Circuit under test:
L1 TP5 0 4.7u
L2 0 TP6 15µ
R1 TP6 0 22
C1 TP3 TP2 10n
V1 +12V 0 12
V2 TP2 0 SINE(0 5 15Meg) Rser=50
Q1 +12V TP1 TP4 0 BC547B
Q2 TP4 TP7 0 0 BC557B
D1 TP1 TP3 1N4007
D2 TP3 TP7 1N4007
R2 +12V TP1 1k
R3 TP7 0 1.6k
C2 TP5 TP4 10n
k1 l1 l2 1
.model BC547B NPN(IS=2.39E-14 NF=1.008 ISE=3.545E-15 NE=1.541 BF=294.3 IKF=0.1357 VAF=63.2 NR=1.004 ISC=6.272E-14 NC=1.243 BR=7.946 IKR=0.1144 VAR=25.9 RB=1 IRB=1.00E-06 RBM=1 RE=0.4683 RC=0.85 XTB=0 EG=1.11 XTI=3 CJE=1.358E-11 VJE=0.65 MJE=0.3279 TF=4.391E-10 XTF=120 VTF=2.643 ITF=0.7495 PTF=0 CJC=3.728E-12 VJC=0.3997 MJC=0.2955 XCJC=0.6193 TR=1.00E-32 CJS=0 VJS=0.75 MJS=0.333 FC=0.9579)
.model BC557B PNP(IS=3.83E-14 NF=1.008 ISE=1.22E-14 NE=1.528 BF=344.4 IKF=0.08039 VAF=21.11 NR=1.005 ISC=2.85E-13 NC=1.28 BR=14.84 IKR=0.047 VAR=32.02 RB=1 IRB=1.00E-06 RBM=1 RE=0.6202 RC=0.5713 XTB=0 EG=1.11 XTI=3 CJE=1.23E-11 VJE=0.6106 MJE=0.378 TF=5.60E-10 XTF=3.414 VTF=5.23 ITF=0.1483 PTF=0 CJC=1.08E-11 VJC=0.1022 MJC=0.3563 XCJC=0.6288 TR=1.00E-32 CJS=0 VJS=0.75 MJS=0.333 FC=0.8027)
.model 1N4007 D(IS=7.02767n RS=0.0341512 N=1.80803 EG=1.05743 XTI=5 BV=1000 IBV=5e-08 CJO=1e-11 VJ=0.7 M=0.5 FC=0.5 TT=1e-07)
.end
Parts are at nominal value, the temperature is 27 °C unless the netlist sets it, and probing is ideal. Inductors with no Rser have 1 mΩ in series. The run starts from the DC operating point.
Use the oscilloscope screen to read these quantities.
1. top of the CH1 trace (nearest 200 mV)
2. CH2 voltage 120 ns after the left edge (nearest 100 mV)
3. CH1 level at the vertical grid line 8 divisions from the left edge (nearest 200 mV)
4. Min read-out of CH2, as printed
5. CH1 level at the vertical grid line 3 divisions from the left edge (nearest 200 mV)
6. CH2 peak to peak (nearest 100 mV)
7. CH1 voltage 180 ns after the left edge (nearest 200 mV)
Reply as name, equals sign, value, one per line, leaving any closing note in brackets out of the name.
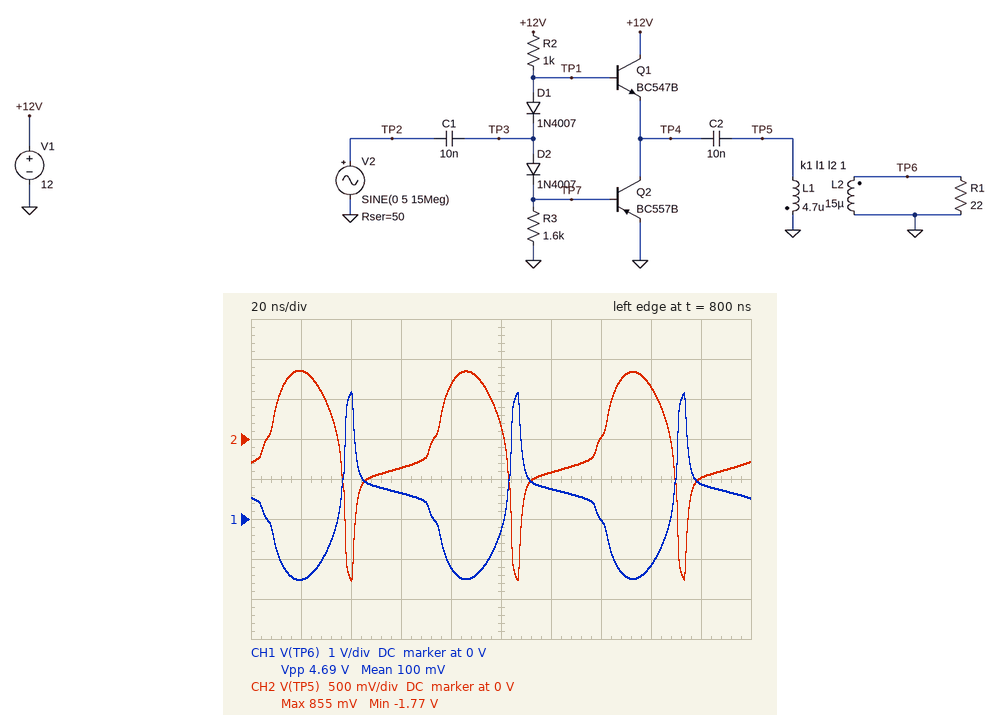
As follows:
top of the CH1 trace = 3.2 V
CH2 voltage 120 ns after the left edge = -400 mV
CH1 level at the vertical grid line 8 divisions from the left edge = -1.2 V
Min read-out of CH2, as printed = -1.77 V
CH1 level at the vertical grid line 3 divisions from the left edge = 600 mV
CH2 peak to peak = 2.6 V
CH1 voltage 180 ns after the left edge = 800 mV
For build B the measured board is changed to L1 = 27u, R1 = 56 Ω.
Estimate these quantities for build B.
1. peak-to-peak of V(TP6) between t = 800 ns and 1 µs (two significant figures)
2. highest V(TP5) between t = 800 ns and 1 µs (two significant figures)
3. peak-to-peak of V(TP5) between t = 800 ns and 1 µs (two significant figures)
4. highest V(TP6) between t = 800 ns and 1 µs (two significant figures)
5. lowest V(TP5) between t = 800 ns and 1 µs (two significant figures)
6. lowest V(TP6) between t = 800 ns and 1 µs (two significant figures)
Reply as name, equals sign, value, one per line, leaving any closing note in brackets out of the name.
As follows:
peak-to-peak of V(TP6) between t = 800 ns and 1 µs = 6.4 V
highest V(TP5) between t = 800 ns and 1 µs = 4.3 V
peak-to-peak of V(TP5) between t = 800 ns and 1 µs = 8.6 V
highest V(TP6) between t = 800 ns and 1 µs = 3.2 V
lowest V(TP5) between t = 800 ns and 1 µs = -4.3 V
lowest V(TP6) between t = 800 ns and 1 µs = -3.2 V
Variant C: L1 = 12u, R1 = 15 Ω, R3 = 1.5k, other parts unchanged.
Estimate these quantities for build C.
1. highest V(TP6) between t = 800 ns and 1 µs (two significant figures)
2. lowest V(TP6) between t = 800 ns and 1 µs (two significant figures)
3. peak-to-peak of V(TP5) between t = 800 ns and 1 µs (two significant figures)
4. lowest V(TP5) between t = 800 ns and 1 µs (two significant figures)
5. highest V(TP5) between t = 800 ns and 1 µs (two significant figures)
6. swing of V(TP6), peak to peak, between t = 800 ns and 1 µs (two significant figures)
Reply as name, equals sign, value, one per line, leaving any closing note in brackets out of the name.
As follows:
highest V(TP6) between t = 800 ns and 1 µs = 2.8 V
lowest V(TP6) between t = 800 ns and 1 µs = -1.6 V
peak-to-peak of V(TP5) between t = 800 ns and 1 µs = 3.9 V
lowest V(TP5) between t = 800 ns and 1 µs = -2.5 V
highest V(TP5) between t = 800 ns and 1 µs = 1.4 V
swing of V(TP6), peak to peak, between t = 800 ns and 1 µs = 4.4 V
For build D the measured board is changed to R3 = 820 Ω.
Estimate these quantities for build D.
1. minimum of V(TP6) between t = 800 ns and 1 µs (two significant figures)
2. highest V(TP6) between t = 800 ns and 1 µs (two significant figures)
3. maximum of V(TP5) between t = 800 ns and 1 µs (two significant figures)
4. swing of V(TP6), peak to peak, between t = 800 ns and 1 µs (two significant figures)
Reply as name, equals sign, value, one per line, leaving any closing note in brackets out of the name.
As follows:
minimum of V(TP6) between t = 800 ns and 1 µs = -1.8 V
highest V(TP6) between t = 800 ns and 1 µs = 3.3 V
maximum of V(TP5) between t = 800 ns and 1 µs = 1.0 V
swing of V(TP6), peak to peak, between t = 800 ns and 1 µs = 5.1 V
